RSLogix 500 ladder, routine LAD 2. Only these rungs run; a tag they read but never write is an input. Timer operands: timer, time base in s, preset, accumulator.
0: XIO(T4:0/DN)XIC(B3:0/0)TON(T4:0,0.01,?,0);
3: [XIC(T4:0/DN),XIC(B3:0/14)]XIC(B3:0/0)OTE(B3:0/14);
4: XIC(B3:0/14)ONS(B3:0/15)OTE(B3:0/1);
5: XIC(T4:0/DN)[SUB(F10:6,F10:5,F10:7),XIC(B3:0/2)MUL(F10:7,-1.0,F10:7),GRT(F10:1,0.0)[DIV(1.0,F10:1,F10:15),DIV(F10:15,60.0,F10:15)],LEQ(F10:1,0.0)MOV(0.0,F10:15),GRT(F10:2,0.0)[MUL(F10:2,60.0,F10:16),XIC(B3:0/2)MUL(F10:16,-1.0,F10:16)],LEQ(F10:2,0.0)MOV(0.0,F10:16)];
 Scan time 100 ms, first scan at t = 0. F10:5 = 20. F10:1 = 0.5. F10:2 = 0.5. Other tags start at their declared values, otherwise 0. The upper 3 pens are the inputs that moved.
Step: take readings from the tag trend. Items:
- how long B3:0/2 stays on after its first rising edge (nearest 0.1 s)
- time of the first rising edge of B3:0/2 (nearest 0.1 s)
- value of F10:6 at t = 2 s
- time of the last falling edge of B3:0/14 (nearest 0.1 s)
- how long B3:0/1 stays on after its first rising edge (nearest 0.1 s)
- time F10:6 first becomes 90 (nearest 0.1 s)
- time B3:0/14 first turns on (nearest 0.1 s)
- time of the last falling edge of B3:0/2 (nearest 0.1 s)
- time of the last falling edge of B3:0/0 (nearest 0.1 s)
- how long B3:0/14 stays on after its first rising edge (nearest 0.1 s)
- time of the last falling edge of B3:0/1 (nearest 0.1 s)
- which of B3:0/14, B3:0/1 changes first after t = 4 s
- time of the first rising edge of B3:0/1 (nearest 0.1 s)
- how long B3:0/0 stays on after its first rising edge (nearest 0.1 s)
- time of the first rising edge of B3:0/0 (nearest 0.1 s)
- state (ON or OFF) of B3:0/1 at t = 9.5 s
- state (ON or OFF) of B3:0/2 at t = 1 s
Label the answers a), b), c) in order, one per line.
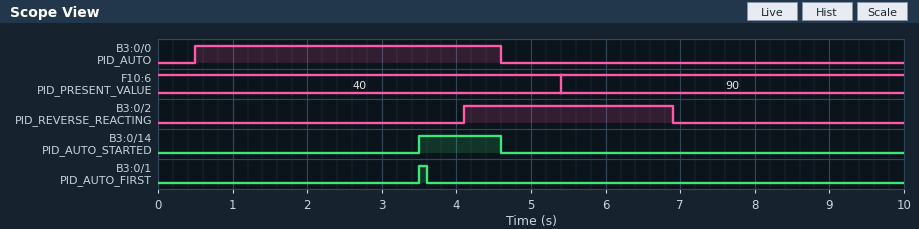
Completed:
a) 2.8 s
b) 4.1 s
c) 40
d) 4.6 s
e) 0.1 s
f) 5.4 s
g) 3.5 s
h) 6.9 s
i) 4.6 s
j) 1.1 s
k) 3.6 s
l) B3:0/14
m) 3.5 s
n) 4.1 s
o) 0.5 s
p) OFF
q) OFF
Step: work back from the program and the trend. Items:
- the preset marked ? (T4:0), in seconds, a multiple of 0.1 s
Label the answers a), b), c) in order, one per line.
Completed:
a) 3.0 s
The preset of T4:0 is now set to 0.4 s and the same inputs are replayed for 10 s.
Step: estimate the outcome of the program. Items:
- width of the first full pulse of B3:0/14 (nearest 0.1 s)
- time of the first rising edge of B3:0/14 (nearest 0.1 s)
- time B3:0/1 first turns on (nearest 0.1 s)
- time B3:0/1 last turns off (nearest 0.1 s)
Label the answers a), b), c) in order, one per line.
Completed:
a) 3.7 s
b) 0.9 s
c) 0.9 s
d) 1.0 s
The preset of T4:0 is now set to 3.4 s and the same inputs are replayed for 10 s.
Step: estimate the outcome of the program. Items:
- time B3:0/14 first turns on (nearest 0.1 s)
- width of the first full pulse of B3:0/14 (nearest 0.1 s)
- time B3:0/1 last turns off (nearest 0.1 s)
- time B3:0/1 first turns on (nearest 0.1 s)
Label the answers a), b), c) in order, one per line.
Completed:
a) 3.9 s
b) 0.7 s
c) 4.0 s
d) 3.9 s
